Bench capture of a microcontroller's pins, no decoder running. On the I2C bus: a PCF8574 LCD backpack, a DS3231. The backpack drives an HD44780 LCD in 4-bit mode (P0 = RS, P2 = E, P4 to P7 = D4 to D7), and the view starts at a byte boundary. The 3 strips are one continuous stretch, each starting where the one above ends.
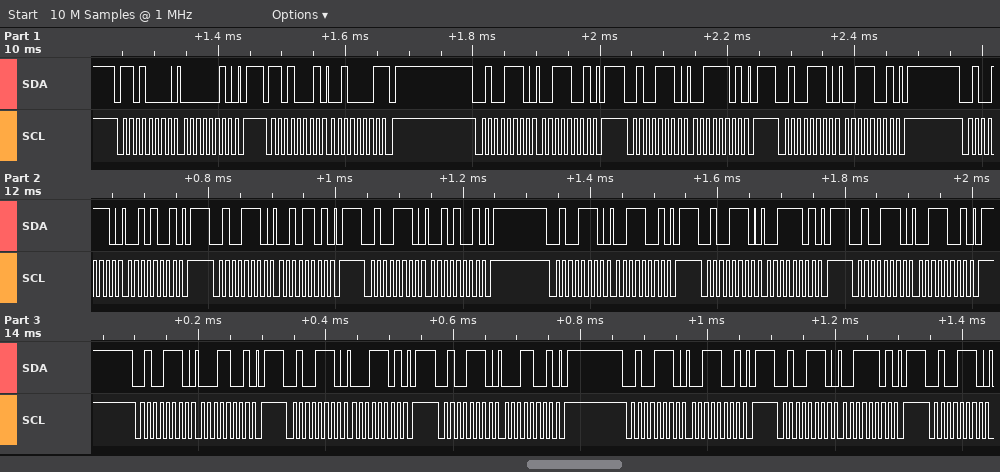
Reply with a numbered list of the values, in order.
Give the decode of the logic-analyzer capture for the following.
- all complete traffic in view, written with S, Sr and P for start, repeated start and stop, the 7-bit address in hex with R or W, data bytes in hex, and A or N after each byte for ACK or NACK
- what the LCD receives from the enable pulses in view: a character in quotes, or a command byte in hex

1. S 68W A 02 A P S 68R A 21 N P S 27W A 39 A P S 27W A 3D A P S 27W A 39 A P S 27W A 29 A P S 27W A 2D A P S 27W A 29 A P S 27W A 39 A P S 27W A 3D A P S 27W A 39 A P S 27W A 19 A P S 27W A 1D A P S 27W A 19 A P S 27W A 39 A P S 27W A 3D A P S 27W A
2. '2' '1'
